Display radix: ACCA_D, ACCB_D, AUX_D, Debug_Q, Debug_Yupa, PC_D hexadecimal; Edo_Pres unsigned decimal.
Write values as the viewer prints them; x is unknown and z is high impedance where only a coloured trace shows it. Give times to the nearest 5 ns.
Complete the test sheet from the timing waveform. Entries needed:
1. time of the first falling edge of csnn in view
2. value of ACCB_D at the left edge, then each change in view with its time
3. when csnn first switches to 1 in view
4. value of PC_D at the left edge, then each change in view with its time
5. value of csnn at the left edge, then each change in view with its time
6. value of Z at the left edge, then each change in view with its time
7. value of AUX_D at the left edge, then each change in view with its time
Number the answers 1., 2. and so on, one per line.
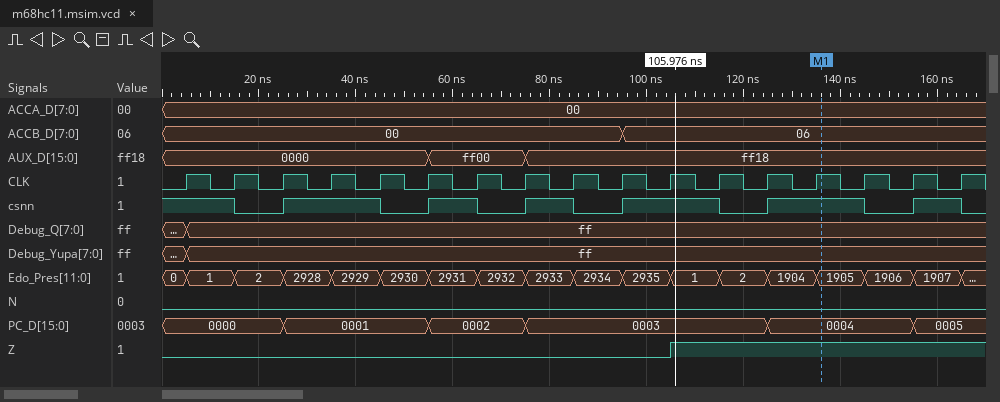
1. 15 ns
2. 00, 06 at 95 ns
3. 25 ns
4. 0000, 0001 at 25 ns, 0002 at 55 ns, 0003 at 75 ns, 0004 at 125 ns, 0005 at 155 ns
5. 1, 0 at 15 ns, 1 at 25 ns, 0 at 45 ns, 1 at 55 ns, 0 at 65 ns, 1 at 75 ns, 0 at 85 ns, 1 at 95 ns, 0 at 115 ns, 1 at 125 ns, 0 at 145 ns, 1 at 155 ns, 0 at 165 ns
6. 0, 1 at 105 ns
7. 0000, ff00 at 55 ns, ff18 at 75 ns
